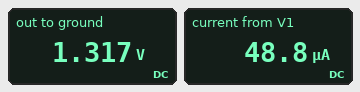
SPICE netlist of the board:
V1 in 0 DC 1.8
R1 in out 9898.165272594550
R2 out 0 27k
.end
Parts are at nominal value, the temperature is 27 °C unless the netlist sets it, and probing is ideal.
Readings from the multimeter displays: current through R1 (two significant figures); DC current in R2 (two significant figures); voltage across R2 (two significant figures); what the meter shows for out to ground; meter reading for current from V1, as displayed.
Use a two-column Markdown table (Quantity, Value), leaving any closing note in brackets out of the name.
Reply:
| Quantity | Value |
|---|---|
| current through R1 | 49 µA |
| DC current in R2 | 49 µA |
| voltage across R2 | 1.3 V |
| what the meter shows for out to ground | 1.317 V |
| meter reading for current from V1, as displayed | 48.8 µA |
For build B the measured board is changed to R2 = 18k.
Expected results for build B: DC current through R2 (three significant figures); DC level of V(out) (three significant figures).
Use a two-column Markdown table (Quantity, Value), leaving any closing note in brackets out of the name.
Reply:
| Quantity | Value |
|---|---|
| DC current through R2 | 64.5 µA |
| DC level of V(out) | 1.16 V |
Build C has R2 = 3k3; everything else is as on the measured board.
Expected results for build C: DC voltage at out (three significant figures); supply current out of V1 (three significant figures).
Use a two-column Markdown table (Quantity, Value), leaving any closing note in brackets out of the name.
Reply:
| Quantity | Value |
|---|---|
| DC voltage at out | 450 mV |
| supply current out of V1 | 136 µA |
